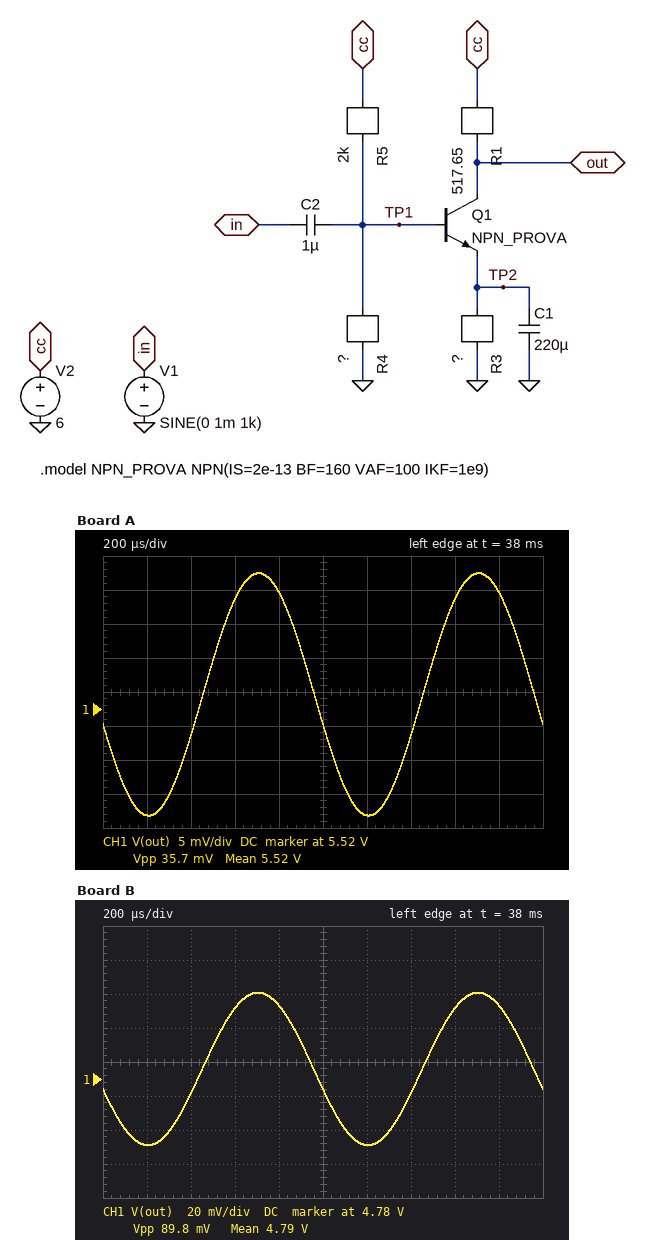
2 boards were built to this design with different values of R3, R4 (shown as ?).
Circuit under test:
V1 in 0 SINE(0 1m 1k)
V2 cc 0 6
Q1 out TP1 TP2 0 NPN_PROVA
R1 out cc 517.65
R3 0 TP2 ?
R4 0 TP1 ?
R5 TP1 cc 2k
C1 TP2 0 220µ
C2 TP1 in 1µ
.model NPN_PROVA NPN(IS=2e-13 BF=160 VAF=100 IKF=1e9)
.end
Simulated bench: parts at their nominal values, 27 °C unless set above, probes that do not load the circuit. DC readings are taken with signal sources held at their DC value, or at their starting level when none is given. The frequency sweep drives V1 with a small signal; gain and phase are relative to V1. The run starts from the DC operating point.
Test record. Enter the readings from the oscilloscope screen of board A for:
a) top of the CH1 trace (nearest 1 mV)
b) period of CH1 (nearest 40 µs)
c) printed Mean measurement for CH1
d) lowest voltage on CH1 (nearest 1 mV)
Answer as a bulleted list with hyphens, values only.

- 5.540 V
- 1.00 ms
- 5.52 V
- 5.504 V
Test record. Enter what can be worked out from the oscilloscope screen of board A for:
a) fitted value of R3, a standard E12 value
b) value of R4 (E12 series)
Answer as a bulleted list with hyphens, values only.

- 1.8 kΩ
- 1.2 kΩ
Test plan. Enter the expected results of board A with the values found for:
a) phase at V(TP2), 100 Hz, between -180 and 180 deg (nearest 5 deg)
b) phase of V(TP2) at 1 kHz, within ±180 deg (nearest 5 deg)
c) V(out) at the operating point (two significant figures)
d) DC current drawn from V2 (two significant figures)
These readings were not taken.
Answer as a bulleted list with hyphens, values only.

- -10 deg
- -75 deg
- 5.5 V
- 2.8 mA
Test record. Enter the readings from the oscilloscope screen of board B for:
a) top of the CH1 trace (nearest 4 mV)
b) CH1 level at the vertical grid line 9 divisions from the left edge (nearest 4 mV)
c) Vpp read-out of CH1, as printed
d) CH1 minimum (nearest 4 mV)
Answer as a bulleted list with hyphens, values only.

- 4.832 V
- 4.824 V
- 89.8 mV
- 4.740 V
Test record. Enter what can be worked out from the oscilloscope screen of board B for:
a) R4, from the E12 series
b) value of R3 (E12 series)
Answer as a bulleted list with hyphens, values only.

- 2.7 kΩ
- 1.2 kΩ
